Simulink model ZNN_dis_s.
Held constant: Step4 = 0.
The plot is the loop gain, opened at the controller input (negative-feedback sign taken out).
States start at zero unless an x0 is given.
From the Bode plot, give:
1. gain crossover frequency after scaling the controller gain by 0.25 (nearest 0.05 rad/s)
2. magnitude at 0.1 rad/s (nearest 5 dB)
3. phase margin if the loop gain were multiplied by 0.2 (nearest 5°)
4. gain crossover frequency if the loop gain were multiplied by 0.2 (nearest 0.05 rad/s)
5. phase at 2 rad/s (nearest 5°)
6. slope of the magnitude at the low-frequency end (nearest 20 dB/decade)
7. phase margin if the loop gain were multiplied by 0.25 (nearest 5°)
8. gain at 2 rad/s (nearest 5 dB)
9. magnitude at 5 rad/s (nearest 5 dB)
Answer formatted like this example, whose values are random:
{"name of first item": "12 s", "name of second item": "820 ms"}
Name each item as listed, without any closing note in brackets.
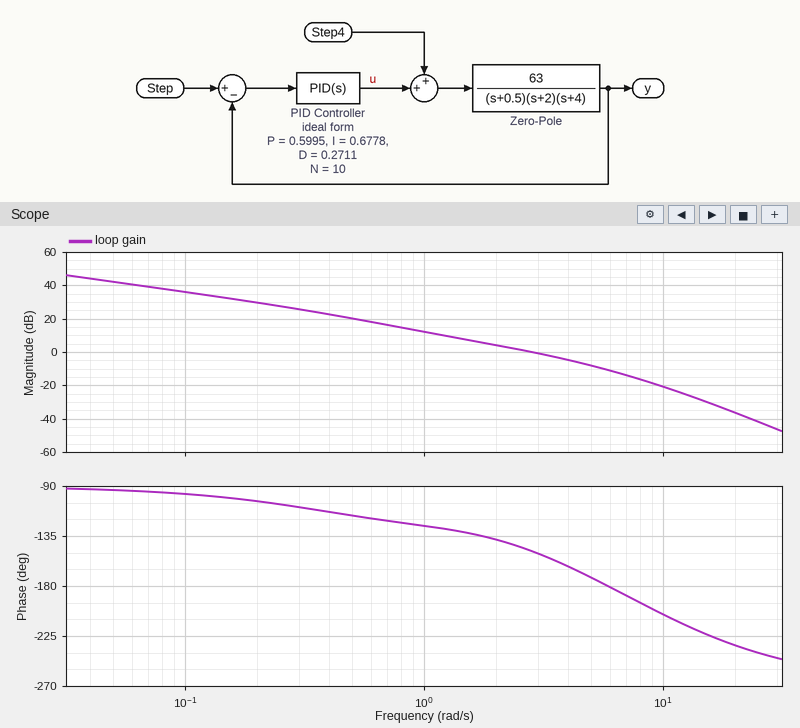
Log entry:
{"gain crossover frequency after scaling the controller gain by 0.25": "1.00 rad/s", "magnitude at 0.1 rad/s": "35 dB", "phase margin if the loop gain were multiplied by 0.2": "55°", "gain crossover frequency if the loop gain were multiplied by 0.2": "0.85 rad/s", "phase at 2 rad/s": "-140°", "slope of the magnitude at the low-frequency end": "-20 dB/decade", "phase margin if the loop gain were multiplied by 0.25": "55°", "gain at 2 rad/s": "5 dB", "magnitude at 5 rad/s": "-10 dB"}
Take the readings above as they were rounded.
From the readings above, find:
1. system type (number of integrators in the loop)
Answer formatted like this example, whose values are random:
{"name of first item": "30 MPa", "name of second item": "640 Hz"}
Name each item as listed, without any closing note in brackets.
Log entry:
{"system type": "1"}
